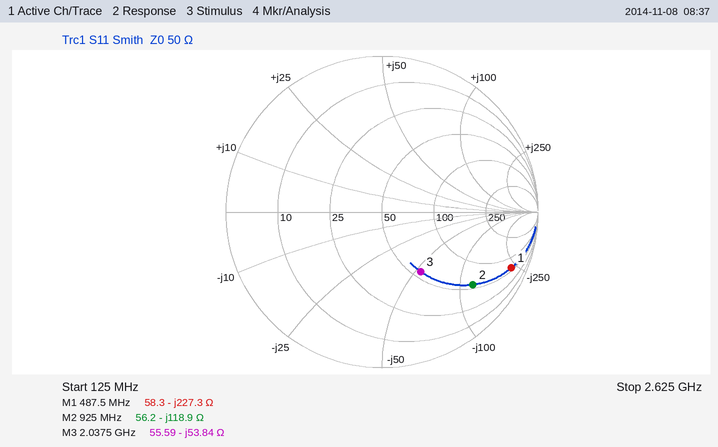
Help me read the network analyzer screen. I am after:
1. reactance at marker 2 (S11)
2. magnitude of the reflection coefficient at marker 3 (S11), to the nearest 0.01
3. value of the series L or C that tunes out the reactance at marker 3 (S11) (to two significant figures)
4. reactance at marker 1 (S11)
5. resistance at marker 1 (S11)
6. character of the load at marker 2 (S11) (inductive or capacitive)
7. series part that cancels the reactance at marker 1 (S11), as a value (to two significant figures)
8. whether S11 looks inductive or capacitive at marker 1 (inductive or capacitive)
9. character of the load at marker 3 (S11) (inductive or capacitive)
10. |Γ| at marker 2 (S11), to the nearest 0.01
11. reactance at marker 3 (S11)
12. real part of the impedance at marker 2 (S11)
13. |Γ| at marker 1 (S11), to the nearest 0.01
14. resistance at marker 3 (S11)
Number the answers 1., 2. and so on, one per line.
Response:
1. -118.9 Ω
2. 0.46
3. 4.2 nH
4. -227.3 Ω
5. 58.3 Ω
6. capacitive
7. 74 nH
8. capacitive
9. capacitive
10. 0.75
11. -53.84 Ω
12. 56.2 Ω
13. 0.90
14. 55.59 Ω
